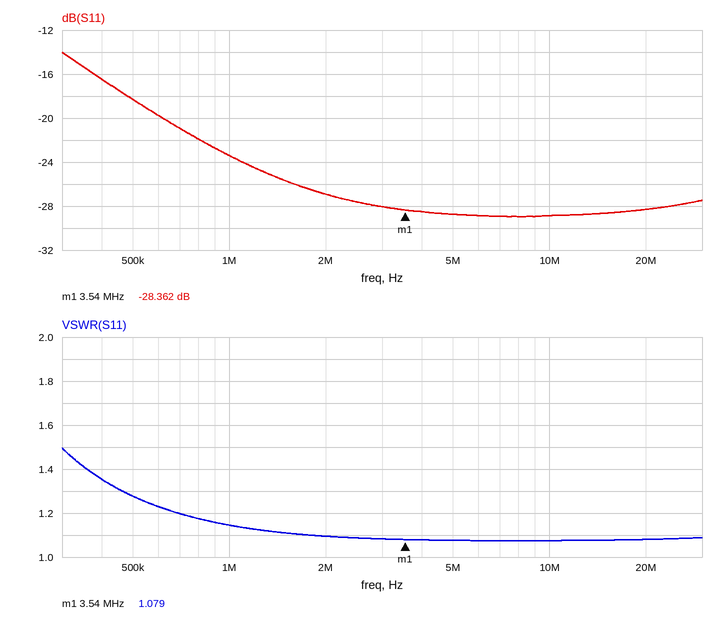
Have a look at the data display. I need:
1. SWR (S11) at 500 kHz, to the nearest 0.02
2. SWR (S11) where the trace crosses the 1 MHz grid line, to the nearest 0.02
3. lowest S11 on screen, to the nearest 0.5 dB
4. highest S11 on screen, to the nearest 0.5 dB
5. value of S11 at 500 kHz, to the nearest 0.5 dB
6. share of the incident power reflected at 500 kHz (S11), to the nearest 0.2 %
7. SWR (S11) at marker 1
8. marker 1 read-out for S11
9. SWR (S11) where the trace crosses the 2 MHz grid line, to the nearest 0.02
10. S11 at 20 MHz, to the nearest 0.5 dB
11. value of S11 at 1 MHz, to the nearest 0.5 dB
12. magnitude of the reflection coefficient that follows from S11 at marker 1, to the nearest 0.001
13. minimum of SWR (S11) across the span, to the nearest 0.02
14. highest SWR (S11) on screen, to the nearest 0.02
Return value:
1.28
1.14
-29.0 dB
-14.0 dB
-18.5 dB
1.4 %
1.079
-28.362 dB
1.10
-28.5 dB
-23.5 dB
0.038
1.08
1.50
